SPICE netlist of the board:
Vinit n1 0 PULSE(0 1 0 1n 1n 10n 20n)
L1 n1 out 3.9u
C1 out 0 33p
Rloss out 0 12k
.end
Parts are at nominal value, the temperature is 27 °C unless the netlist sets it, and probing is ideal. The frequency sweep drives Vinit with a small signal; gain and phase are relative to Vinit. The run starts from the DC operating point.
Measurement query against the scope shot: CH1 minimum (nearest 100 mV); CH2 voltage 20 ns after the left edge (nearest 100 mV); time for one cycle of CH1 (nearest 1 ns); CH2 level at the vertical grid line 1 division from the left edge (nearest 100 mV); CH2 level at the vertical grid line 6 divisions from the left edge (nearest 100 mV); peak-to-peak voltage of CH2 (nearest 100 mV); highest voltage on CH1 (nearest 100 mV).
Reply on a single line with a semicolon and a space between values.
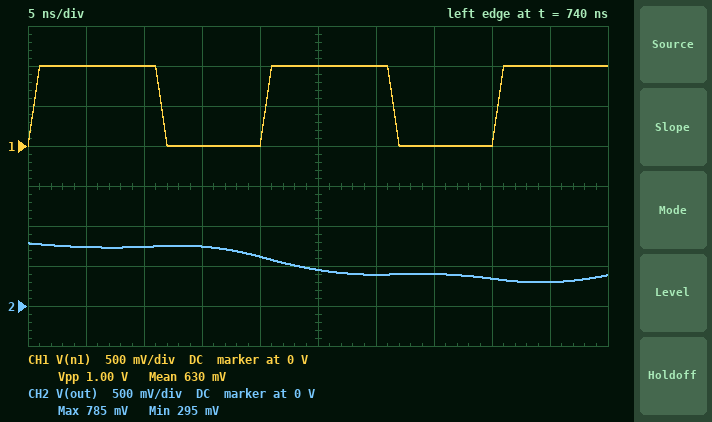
0 V; 600 mV; 20 ns; 700 mV; 400 mV; 500 mV; 1.0 V
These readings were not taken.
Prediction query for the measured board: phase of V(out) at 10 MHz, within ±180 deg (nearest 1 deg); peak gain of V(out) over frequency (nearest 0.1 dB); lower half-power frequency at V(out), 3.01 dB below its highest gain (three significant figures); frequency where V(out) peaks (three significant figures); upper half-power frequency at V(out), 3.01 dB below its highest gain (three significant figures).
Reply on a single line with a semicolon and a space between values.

-2 deg; 30.9 dB; 13.8 MHz; 14.0 MHz; 14.2 MHz
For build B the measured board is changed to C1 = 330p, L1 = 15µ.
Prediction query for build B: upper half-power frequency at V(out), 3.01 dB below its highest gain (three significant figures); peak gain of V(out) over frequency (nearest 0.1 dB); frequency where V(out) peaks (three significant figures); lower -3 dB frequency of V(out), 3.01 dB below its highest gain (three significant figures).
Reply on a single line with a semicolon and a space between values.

2.28 MHz; 35.0 dB; 2.26 MHz; 2.24 MHz
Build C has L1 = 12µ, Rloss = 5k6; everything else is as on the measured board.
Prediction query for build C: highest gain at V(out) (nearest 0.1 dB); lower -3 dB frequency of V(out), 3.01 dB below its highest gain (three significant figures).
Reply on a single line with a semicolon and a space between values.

19.4 dB; 7.53 MHz
